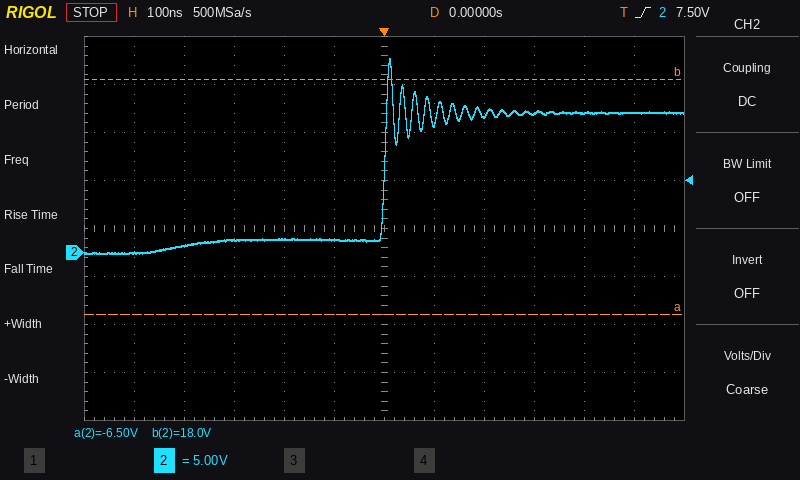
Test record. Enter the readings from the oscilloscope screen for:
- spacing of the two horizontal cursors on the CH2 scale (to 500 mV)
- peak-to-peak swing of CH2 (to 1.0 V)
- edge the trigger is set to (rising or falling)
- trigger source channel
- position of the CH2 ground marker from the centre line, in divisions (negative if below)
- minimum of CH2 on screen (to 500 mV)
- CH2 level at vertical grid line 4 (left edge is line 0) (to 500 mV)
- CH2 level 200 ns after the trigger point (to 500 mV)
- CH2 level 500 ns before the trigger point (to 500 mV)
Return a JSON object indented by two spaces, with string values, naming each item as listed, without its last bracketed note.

{
  "spacing of the two horizontal cursors on the CH2 scale": "24.5 V",
  "peak-to-peak swing of CH2": "20.0 V",
  "edge the trigger is set to": "rising",
  "trigger source channel": "CH2",
  "position of the CH2 ground marker from the centre line, in divisions": "-0.5 div",
  "minimum of CH2 on screen": "0.0 V",
  "CH2 level at vertical grid line 4 (left edge is line 0)": "1.5 V",
  "CH2 level 200 ns after the trigger point": "14.5 V",
  "CH2 level 500 ns before the trigger point": "0.0 V"
}
